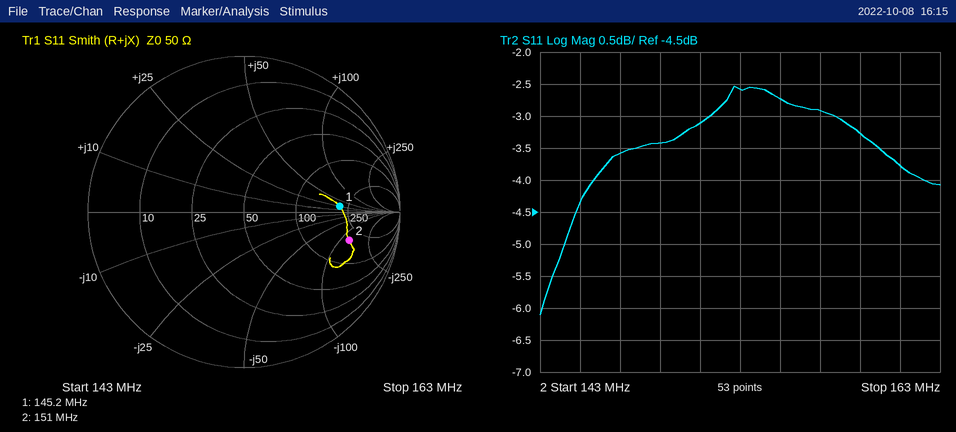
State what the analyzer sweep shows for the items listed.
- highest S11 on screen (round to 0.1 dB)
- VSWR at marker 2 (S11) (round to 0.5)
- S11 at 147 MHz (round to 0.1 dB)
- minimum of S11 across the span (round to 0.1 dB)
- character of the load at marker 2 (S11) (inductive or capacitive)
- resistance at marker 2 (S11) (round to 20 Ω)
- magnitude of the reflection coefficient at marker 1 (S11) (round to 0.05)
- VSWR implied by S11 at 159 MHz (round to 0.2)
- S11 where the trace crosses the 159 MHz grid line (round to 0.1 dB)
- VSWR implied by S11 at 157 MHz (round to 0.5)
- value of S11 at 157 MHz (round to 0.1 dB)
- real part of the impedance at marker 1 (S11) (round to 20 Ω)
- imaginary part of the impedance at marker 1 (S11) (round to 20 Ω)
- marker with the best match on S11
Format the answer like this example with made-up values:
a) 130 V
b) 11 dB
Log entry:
a) -2.5 dB
b) 5.5
c) -3.6 dB
d) -6.1 dB
e) capacitive
f) 180 Ω
g) 0.60
h) 5.4
i) -3.3 dB
j) 6.0
k) -2.9 dB
l) 200 Ω
m) +20 Ω
n) marker 1
